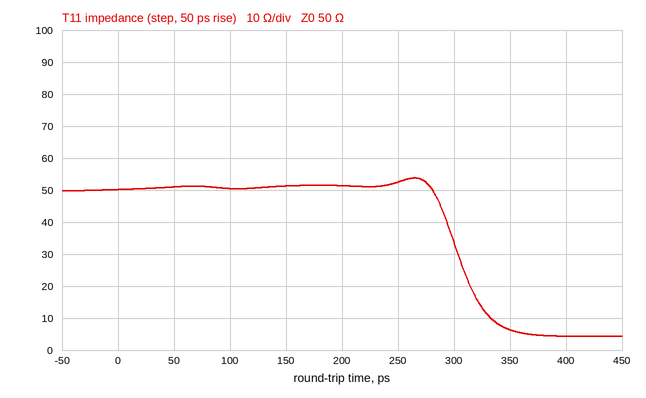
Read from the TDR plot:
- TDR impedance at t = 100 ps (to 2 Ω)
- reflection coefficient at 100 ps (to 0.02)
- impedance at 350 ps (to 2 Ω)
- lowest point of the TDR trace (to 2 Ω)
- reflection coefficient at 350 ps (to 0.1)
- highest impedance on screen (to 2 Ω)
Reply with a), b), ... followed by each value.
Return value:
a) 50 Ω
b) 0.00
c) 6 Ω
d) 4 Ω
e) -0.8
f) 54 Ω
